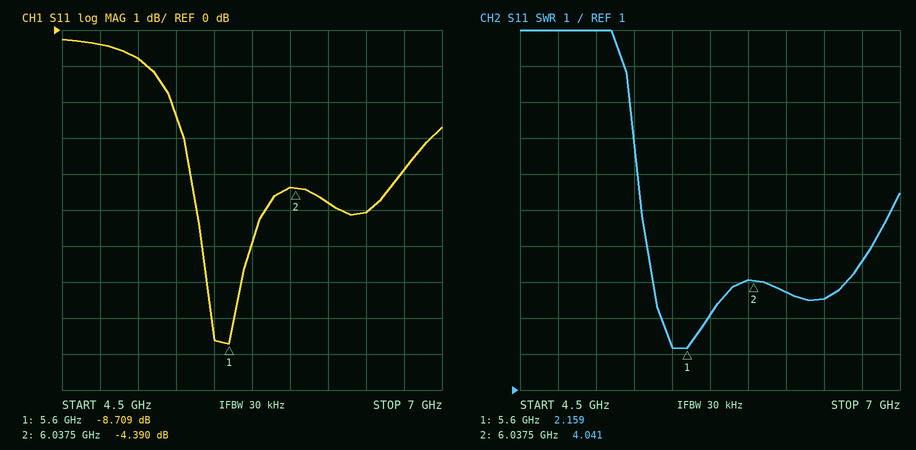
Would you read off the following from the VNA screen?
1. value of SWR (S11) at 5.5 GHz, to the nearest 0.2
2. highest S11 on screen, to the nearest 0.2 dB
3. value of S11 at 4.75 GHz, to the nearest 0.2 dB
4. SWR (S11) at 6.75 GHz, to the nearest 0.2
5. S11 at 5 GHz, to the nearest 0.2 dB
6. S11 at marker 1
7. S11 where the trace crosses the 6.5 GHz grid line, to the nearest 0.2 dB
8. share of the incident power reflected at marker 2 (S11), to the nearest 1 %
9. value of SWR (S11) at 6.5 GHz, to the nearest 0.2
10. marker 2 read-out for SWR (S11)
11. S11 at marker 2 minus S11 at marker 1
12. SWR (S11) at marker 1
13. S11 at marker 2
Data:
2.2
-0.2 dB
-0.4 dB
4.6
-0.8 dB
-8.709 dB
-5.0 dB
36 %
3.6
4.041
4.319 dB
2.159
-4.390 dB
